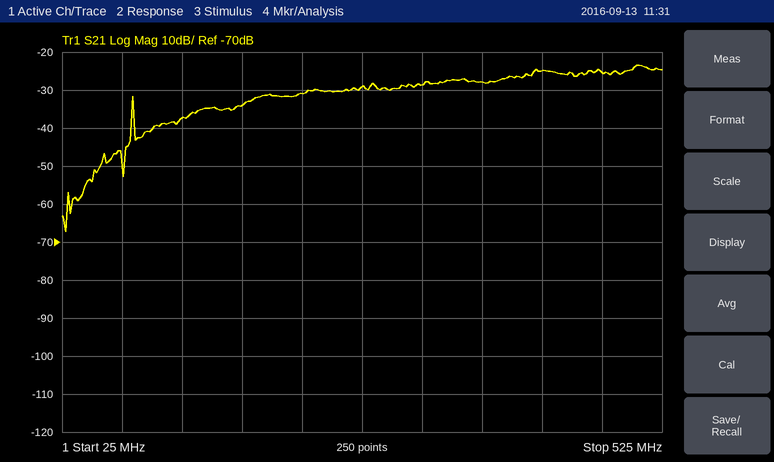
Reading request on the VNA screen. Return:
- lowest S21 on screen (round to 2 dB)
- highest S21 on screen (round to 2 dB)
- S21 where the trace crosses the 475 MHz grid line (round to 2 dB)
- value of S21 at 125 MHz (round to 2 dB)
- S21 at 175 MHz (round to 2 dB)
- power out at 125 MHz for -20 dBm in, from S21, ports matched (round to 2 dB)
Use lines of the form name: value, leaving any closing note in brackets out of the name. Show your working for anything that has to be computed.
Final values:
lowest S21 on screen: -68 dB
highest S21 on screen: -24 dB
S21 where the trace crosses the 475 MHz grid line: -26 dB
value of S21 at 125 MHz: -38 dB
S21 at 175 MHz: -34 dB
power out at 125 MHz for -20 dBm in, from S21, ports matched: -20 dBm + (-38 dB) = -58 dBm
